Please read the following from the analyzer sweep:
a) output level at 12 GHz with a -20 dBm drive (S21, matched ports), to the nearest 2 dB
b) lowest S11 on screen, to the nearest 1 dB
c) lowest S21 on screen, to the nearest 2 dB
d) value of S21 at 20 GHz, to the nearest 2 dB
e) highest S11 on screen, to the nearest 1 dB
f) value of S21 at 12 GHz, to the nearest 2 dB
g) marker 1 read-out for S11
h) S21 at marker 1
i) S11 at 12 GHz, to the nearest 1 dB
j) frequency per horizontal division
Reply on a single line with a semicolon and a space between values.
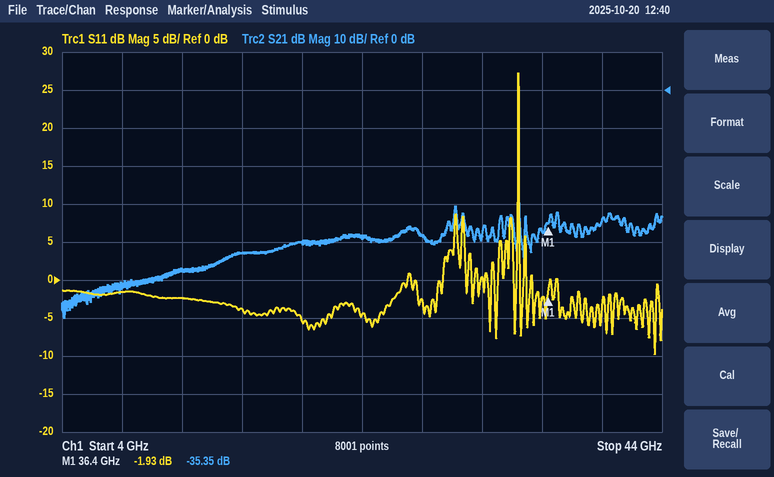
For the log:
-68 dBm; -10 dB; -60 dB; -40 dB; 27 dB; -48 dB; -1.93 dB; -35.35 dB; -2 dB; 4 GHz
